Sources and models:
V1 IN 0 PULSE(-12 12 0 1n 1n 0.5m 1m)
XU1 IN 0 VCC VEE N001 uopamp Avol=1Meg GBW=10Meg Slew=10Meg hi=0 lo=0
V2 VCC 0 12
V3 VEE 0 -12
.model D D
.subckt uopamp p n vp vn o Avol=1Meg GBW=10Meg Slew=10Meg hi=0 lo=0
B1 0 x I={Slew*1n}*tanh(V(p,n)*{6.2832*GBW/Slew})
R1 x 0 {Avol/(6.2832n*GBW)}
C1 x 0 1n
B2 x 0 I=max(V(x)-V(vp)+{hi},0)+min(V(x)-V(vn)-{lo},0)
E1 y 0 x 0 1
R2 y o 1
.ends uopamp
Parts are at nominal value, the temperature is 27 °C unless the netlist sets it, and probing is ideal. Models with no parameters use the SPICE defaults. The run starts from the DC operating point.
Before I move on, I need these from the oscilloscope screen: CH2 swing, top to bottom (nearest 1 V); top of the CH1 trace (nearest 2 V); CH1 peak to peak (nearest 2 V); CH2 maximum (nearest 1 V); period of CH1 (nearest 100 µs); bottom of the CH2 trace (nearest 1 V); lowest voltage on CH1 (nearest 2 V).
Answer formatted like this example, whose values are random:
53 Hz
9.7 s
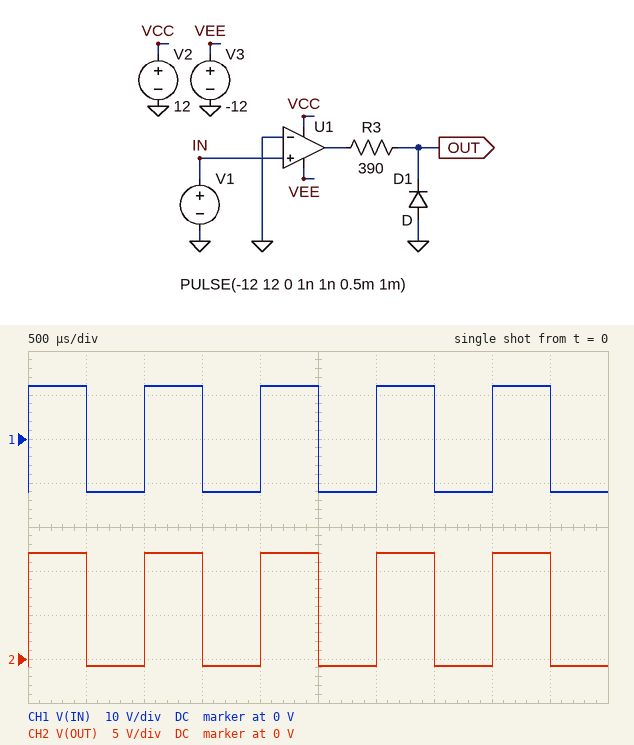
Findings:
13 V
12 V
24 V
12 V
1.0 ms
-1 V
-12 V
